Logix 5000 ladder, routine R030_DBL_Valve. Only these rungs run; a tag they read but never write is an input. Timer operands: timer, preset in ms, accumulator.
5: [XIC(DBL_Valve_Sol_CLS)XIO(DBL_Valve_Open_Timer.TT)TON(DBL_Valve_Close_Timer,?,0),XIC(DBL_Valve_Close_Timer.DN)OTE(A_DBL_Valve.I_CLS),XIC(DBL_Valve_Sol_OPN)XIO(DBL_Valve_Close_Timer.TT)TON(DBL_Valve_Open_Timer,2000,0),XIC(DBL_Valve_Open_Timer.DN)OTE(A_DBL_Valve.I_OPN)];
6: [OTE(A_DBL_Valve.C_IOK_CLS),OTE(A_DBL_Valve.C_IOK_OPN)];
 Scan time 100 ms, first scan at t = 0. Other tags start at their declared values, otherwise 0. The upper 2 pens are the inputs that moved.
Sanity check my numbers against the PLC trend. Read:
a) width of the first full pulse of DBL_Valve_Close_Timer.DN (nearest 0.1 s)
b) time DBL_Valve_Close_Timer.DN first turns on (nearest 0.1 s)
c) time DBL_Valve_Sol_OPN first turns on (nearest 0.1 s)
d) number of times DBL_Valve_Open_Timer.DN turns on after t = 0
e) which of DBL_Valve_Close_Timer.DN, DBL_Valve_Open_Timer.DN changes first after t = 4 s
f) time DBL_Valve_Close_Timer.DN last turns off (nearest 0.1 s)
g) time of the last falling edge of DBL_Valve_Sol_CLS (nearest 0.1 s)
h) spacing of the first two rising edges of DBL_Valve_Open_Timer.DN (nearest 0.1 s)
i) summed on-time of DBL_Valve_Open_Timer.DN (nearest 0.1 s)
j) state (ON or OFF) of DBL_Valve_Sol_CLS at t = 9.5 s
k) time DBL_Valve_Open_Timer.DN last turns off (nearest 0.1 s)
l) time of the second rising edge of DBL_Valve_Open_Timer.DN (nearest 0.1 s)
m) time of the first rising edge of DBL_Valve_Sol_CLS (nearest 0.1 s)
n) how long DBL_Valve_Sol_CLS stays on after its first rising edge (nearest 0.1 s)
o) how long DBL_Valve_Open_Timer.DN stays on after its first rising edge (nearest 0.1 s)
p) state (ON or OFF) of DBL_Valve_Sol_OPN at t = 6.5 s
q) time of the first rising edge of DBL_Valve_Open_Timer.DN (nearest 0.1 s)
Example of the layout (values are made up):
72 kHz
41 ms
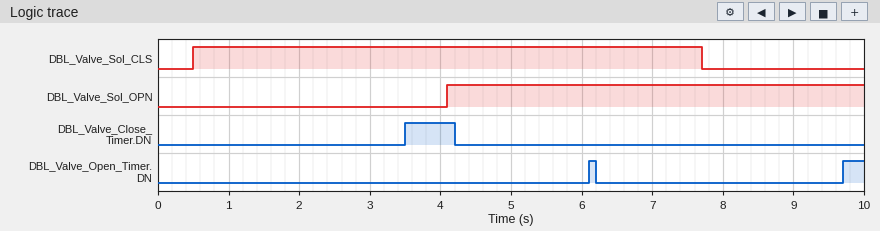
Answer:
0.7 s
3.5 s
4.1 s
2
DBL_Valve_Close_Timer.DN
4.2 s
7.7 s
3.6 s
0.4 s
OFF
6.2 s
9.7 s
0.5 s
7.2 s
0.1 s
ON
6.1 s
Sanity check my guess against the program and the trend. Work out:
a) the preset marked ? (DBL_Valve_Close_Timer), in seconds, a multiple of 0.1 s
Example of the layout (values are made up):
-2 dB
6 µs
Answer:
3.0 s
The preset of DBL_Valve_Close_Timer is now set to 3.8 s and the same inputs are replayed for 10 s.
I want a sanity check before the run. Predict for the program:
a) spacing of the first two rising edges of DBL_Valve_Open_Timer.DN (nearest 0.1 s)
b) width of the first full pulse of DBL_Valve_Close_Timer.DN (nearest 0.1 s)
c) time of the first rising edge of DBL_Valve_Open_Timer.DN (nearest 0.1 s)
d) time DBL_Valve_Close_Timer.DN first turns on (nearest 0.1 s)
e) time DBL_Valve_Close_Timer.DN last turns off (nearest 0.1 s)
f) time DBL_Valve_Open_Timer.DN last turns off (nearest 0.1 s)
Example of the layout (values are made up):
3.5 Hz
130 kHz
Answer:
3.4 s
0.1 s
6.3 s
4.3 s
4.4 s
6.4 s
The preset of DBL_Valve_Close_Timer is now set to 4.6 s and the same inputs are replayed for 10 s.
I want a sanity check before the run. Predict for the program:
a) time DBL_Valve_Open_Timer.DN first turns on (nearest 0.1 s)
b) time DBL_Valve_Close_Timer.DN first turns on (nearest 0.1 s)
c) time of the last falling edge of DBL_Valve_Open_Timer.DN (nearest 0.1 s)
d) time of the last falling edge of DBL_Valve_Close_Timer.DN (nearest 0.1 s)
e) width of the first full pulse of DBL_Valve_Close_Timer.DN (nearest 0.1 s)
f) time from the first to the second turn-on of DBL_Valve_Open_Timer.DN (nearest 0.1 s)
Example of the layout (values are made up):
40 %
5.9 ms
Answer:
7.1 s
5.1 s
7.2 s
5.2 s
0.1 s
2.6 s
